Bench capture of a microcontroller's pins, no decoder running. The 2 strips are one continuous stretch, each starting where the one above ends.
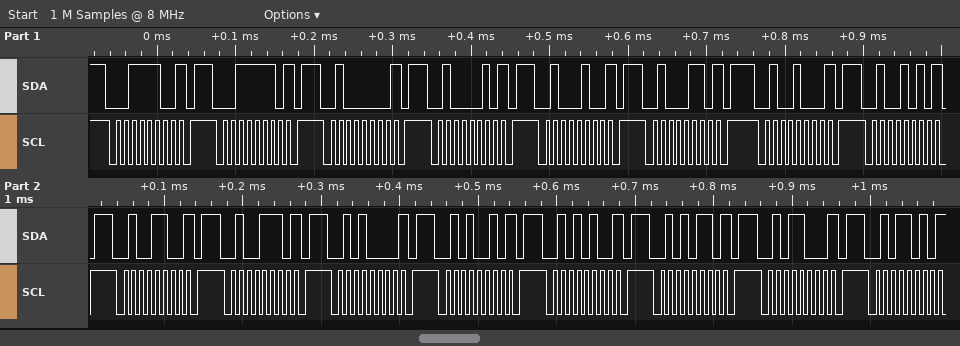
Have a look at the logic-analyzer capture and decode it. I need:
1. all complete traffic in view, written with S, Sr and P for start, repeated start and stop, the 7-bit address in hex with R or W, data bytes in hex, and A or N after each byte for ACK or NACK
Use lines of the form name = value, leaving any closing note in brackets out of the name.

all complete traffic in view, written with S, Sr and P for start, repeated start and stop, the 7-bit address in hex with R or W, data bytes in hex, and A or N after each byte for ACK or NACK = S 1EW N P S 1FW N P S 20W N P S 21W N P S 22W N P S 23W N P S 24W N P S 25W N P S 26W N P S 27W N P S 28W N P S 29W N P S 2AW N P S 2BW N P S 2CW N P S 2DW N
